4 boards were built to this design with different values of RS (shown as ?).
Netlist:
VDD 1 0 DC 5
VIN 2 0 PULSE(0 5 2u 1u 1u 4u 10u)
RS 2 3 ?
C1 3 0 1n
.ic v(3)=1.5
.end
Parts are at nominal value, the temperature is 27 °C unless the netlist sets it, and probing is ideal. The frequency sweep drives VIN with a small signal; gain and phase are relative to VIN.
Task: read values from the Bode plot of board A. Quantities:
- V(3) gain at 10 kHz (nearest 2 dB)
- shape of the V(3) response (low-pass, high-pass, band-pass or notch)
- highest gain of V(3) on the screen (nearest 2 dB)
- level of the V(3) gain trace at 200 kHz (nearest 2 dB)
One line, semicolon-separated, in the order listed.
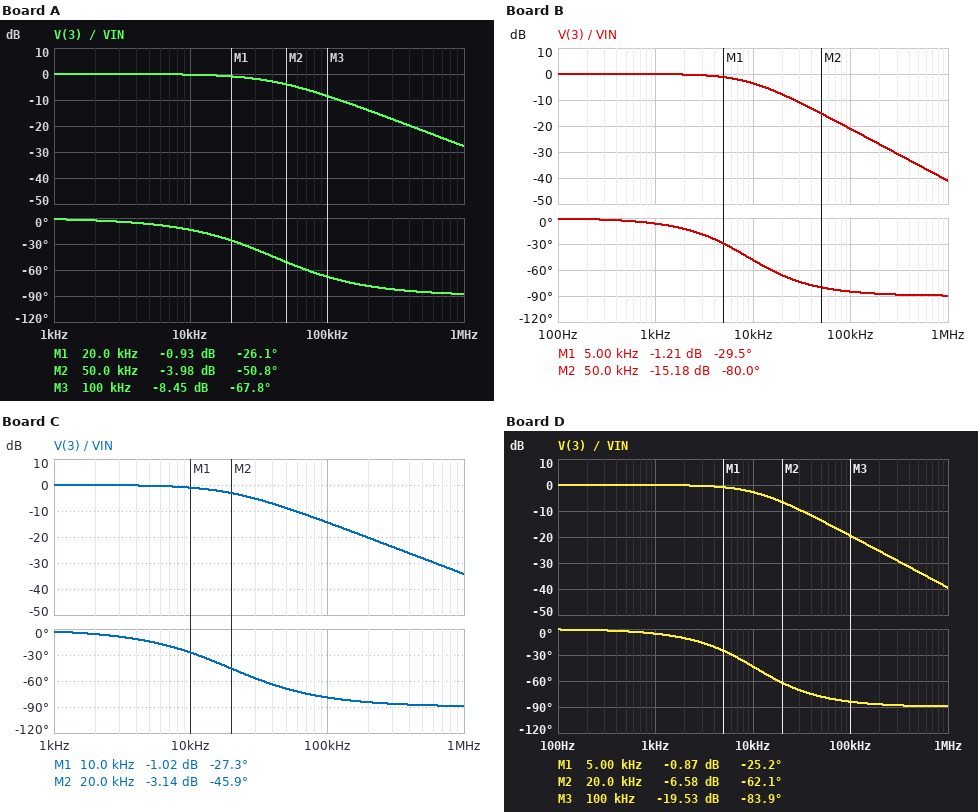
0 dB; low-pass; 0 dB; -14 dB
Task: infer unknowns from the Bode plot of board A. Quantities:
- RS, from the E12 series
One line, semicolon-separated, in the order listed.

3.9 kΩ
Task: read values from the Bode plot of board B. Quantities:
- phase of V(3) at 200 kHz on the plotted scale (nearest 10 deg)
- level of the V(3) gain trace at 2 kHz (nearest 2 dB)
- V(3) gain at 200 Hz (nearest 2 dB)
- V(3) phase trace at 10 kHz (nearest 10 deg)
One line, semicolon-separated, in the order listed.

-90 deg; 0 dB; 0 dB; -50 deg
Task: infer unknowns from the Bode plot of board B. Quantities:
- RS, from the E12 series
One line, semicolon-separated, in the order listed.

18 kΩ
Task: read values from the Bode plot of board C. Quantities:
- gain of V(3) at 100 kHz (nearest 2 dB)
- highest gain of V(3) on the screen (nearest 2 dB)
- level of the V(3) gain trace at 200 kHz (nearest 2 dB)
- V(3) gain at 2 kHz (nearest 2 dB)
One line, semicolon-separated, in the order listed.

-14 dB; 0 dB; -20 dB; 0 dB
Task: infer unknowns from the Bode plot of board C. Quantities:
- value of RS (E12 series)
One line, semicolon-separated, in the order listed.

8.2 kΩ
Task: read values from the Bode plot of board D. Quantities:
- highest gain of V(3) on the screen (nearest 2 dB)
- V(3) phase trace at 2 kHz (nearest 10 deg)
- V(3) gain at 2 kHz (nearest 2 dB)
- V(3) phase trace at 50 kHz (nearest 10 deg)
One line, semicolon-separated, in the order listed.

0 dB; -10 deg; 0 dB; -80 deg
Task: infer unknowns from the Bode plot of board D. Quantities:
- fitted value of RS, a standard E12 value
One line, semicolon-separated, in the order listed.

15 kΩ
